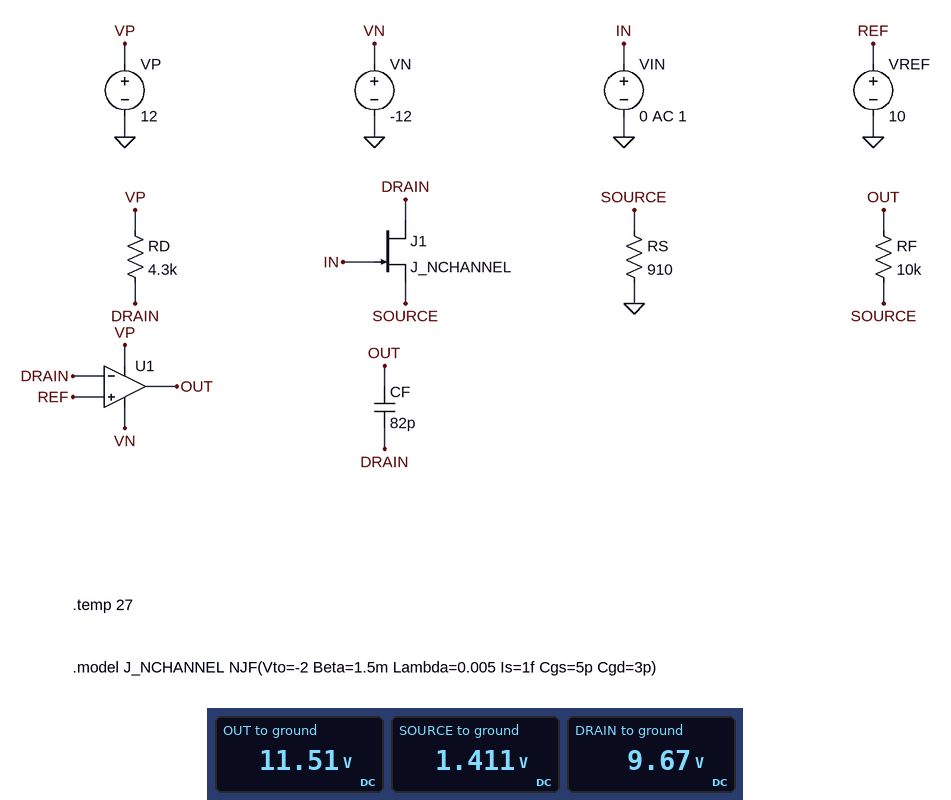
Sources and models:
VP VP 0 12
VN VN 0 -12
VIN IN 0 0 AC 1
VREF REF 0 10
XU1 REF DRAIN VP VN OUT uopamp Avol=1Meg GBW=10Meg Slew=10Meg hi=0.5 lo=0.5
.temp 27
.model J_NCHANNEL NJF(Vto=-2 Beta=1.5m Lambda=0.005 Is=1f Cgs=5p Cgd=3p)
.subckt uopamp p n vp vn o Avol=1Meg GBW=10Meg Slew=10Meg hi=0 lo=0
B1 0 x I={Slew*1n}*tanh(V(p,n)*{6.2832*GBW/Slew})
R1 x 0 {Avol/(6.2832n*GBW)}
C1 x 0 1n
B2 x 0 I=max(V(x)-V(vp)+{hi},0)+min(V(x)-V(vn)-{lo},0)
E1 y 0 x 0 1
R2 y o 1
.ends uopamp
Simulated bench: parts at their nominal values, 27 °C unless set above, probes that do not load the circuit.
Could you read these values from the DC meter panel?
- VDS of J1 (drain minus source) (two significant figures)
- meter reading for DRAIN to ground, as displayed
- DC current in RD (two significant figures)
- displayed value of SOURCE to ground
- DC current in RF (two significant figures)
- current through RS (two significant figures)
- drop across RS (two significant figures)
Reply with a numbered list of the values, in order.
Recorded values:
1. 8.3 V
2. 9.67 V
3. 540 µA
4. 1.411 V
5. 1.0 mA
6. 1.6 mA
7. 1.4 V
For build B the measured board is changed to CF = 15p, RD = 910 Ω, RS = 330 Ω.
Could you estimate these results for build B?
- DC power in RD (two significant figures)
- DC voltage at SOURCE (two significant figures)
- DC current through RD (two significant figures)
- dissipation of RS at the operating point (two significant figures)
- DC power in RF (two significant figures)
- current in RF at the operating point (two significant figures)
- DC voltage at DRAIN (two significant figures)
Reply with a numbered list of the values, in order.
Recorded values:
1. 4.4 mW
2. 820 mV
3. 2.2 mA
4. 2.0 mW
5. 760 µW
6. 280 µA
7. 10 V
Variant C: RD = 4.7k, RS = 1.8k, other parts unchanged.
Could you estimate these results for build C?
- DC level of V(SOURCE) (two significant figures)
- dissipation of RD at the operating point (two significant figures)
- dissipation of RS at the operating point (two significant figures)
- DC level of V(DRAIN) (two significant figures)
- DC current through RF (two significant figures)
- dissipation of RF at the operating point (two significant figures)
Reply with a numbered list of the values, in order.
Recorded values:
1. 1.5 V
2. 850 µW
3. 1.2 mW
4. 10 V
5. 400 µA
6. 1.6 mW
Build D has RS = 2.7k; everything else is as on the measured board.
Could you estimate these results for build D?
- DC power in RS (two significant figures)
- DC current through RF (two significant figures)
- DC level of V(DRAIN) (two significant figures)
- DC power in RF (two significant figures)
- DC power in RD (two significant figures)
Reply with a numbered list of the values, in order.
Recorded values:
1. 780 µW
2. 74 µA
3. 10 V
4. 54 µW
5. 930 µW
